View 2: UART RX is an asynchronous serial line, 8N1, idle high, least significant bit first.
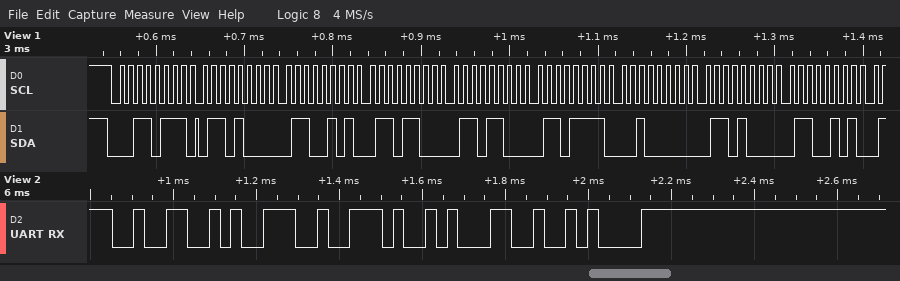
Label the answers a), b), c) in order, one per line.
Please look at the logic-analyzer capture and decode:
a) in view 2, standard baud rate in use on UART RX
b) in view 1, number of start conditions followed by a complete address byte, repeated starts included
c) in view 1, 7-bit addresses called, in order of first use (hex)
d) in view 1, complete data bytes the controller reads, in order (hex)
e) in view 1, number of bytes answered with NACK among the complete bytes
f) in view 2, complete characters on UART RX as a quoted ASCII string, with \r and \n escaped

a) 38400 baud
b) 1
c) 0x1B
d) 68 65 6C 6C 6F 20 68 65
e) 0
f) "29.1\n"
